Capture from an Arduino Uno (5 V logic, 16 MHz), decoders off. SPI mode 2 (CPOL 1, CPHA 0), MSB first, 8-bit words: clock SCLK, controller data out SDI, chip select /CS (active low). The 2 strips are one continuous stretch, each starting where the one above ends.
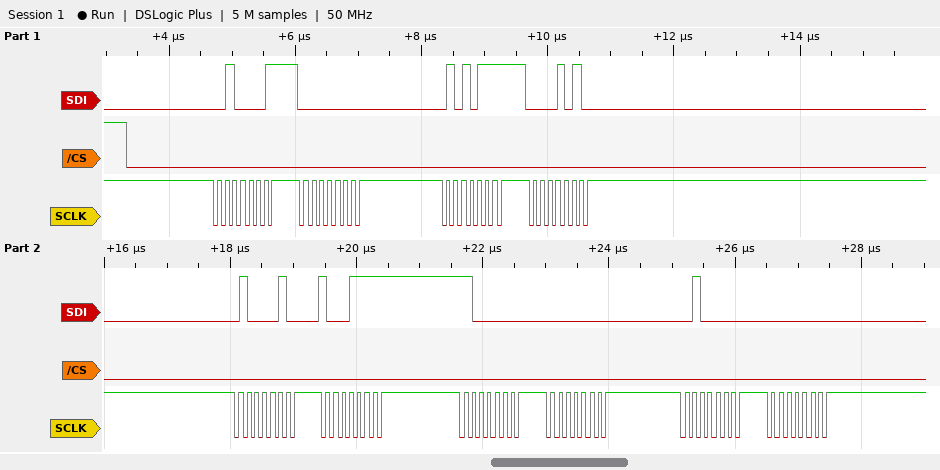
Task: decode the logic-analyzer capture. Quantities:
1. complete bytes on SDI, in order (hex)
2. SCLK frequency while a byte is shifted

21 00 57 0A 42 8F C0 00 20 00
8 MHz
